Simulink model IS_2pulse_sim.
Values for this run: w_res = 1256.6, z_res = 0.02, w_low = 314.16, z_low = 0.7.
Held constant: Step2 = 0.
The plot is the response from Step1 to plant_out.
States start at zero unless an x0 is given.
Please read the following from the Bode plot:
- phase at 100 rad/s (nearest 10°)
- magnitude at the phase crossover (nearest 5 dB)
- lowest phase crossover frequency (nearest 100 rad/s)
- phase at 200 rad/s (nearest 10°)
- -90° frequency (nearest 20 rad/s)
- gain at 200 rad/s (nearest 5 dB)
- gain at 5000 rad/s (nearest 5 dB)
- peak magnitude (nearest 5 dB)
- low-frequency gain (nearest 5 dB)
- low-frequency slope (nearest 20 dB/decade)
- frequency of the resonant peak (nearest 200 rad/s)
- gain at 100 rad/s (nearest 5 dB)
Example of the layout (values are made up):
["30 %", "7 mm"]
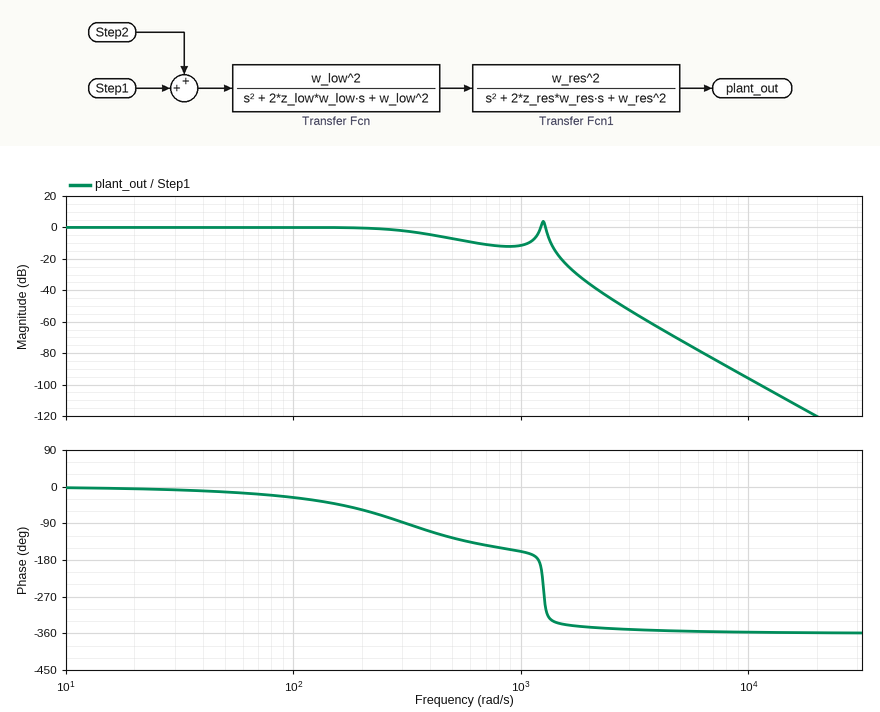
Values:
["-30°", "-5 dB", "1200 rad/s", "-60°", "320 rad/s", "0 dB", "-70 dB", "5 dB", "0 dB", "0 dB/decade", "1200 rad/s", "0 dB"]
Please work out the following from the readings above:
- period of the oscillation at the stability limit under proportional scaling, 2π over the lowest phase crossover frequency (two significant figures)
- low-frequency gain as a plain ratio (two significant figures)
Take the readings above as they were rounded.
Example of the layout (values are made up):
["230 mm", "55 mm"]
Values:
["0.0052 s", "1.0"]
